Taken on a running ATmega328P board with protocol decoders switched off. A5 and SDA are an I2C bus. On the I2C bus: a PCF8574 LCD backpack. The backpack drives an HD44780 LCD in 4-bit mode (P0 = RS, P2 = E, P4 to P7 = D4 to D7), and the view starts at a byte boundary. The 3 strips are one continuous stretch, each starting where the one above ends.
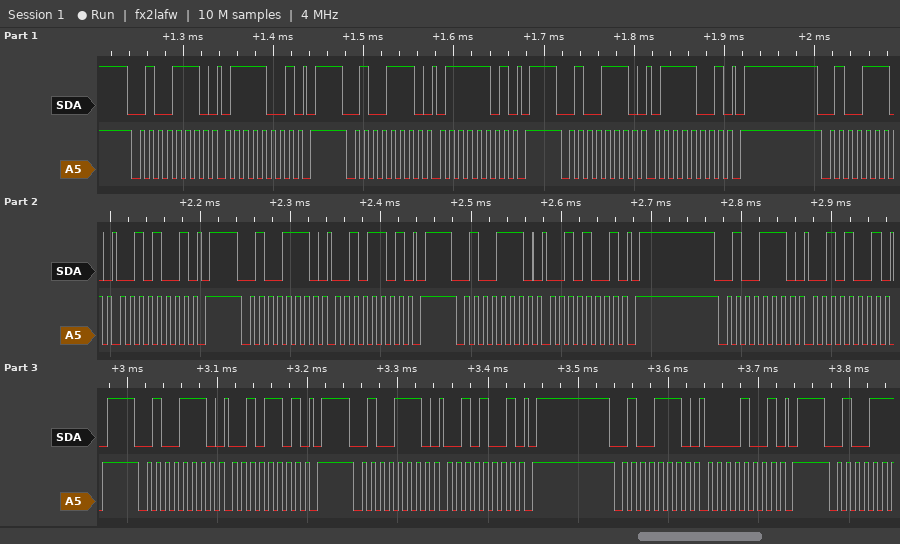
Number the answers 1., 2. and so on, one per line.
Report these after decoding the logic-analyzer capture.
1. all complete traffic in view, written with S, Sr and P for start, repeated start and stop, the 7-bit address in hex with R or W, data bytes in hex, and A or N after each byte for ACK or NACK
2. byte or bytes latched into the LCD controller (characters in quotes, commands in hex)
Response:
1. S 27W A 79 A P S 27W A 7D A P S 27W A 79 A P S 27W A 29 A P S 27W A 2D A P S 27W A 29 A P S 27W A 29 A P S 27W A 2D A P S 27W A 29 A P S 27W A 09 A P
2. 'r'
